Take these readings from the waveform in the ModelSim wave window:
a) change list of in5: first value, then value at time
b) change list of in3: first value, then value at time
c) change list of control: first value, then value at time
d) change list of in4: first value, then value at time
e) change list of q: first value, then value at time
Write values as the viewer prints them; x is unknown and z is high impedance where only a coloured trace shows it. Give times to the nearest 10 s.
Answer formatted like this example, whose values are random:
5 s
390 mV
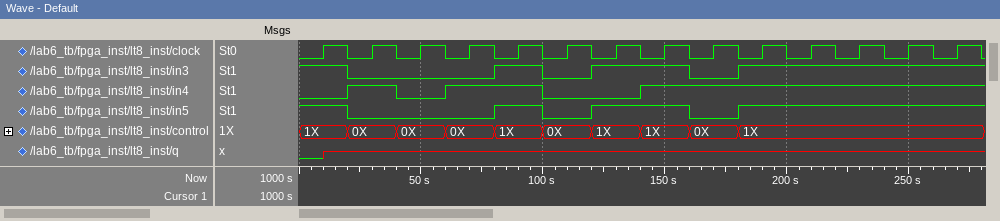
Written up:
1, 0 at 20 s, 1 at 80 s, 0 at 100 s, 1 at 120 s, 0 at 160 s, 1 at 180 s
1, 0 at 20 s, 1 at 80 s, 0 at 100 s, 1 at 120 s, 0 at 160 s, 1 at 180 s
1X, 0X at 20 s, 0X at 40 s, 0X at 60 s, 1X at 80 s, 0X at 100 s, 1X at 120 s, 1X at 140 s, 0X at 160 s, 1X at 180 s
0, 1 at 20 s, 0 at 40 s, 1 at 60 s, 0 at 100 s, 1 at 140 s
0, x at 10 s
